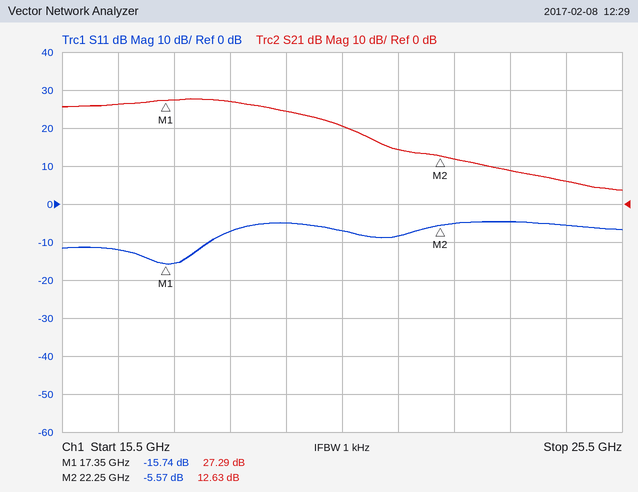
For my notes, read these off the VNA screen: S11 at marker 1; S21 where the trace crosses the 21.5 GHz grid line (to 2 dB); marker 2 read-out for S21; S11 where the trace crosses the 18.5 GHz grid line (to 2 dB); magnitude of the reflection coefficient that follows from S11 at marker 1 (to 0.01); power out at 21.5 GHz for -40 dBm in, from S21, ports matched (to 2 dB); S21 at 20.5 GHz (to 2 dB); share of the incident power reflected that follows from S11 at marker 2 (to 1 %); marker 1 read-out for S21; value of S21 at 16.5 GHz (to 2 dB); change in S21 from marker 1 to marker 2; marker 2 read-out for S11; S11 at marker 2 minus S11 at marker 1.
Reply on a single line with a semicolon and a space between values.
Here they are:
-15.74 dB; 14 dB; 12.63 dB; -8 dB; 0.16; -26 dBm; 20 dB; 28 %; 27.29 dB; 26 dB; -14.66 dB; -5.57 dB; 10.17 dB
